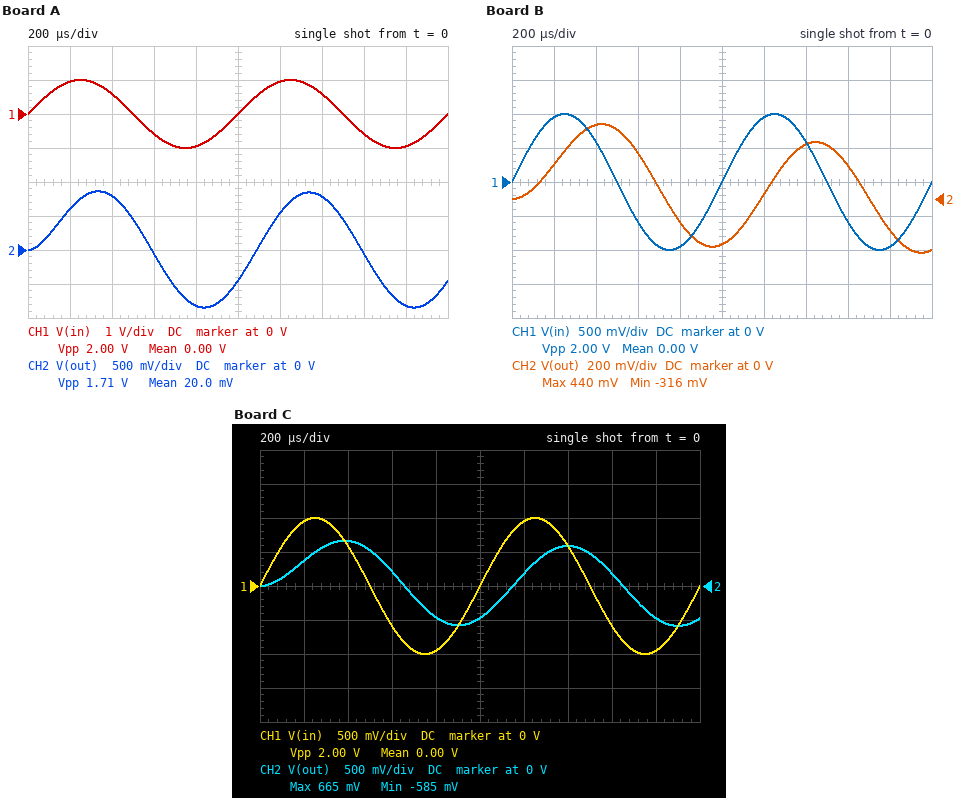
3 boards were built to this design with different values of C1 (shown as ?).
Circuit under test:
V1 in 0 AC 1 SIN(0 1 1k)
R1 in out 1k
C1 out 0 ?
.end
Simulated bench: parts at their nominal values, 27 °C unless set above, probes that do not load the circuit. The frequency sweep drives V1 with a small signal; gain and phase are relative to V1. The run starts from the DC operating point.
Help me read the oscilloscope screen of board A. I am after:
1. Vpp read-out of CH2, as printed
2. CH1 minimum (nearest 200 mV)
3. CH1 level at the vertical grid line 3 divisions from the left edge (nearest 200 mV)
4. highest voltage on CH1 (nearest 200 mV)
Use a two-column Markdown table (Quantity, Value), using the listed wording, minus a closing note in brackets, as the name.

| Quantity | Value |
|---|---|
| Vpp read-out of CH2, as printed | 1.71 V |
| CH1 minimum | -1.0 V |
| CH1 level at the vertical grid line 3 divisions from the left edge | -600 mV |
| highest voltage on CH1 | 1.0 V |
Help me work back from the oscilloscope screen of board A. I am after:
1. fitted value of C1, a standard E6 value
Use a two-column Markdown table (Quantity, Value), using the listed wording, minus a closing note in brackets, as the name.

| Quantity | Value |
|---|---|
| fitted value of C1, a standard E6 value | 100 nF |
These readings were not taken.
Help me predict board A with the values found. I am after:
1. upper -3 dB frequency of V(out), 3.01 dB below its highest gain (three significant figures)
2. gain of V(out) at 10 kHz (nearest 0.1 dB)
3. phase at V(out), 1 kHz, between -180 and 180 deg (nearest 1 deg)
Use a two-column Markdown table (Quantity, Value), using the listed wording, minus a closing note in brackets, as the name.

| Quantity | Value |
|---|---|
| upper -3 dB frequency of V(out), 3.01 dB below its highest gain | 1.59 kHz |
| gain of V(out) at 10 kHz | -16.1 dB |
| phase at V(out), 1 kHz, between -180 and 180 deg | -32 deg |
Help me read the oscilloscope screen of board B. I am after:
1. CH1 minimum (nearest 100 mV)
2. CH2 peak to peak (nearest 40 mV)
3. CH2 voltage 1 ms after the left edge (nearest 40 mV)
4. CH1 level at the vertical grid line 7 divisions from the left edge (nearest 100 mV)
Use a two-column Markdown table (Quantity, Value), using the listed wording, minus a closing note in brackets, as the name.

| Quantity | Value |
|---|---|
| CH1 minimum | -1.0 V |
| CH2 peak to peak | 760 mV |
| CH2 voltage 1 ms after the left edge | -280 mV |
| CH1 level at the vertical grid line 7 divisions from the left edge | 600 mV |
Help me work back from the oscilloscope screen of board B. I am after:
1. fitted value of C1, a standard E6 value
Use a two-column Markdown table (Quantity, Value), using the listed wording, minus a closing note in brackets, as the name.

| Quantity | Value |
|---|---|
| fitted value of C1, a standard E6 value | 470 nF |
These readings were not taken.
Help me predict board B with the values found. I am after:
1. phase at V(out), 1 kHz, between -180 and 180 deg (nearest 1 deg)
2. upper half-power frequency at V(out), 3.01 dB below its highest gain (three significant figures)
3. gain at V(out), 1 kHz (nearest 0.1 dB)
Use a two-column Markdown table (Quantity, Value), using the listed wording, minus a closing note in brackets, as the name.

| Quantity | Value |
|---|---|
| phase at V(out), 1 kHz, between -180 and 180 deg | -71 deg |
| upper half-power frequency at V(out), 3.01 dB below its highest gain | 339 Hz |
| gain at V(out), 1 kHz | -9.9 dB |
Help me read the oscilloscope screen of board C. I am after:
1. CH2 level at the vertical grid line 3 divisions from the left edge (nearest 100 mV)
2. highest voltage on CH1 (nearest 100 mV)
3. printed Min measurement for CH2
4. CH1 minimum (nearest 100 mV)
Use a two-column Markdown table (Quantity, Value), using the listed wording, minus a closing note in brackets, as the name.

| Quantity | Value |
|---|---|
| CH2 level at the vertical grid line 3 divisions from the left edge | 200 mV |
| highest voltage on CH1 | 1.0 V |
| printed Min measurement for CH2 | -585 mV |
| CH1 minimum | -1.0 V |
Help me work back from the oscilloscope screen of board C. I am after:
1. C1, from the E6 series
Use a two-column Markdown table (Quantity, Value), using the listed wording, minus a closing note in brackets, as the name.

| Quantity | Value |
|---|---|
| C1, from the E6 series | 220 nF |
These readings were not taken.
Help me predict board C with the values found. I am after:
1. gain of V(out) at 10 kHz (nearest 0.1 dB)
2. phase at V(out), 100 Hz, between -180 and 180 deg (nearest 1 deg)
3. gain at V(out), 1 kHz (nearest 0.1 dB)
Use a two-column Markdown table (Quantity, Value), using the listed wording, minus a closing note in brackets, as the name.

| Quantity | Value |
|---|---|
| gain of V(out) at 10 kHz | -22.8 dB |
| phase at V(out), 100 Hz, between -180 and 180 deg | -8 deg |
| gain at V(out), 1 kHz | -4.6 dB |
